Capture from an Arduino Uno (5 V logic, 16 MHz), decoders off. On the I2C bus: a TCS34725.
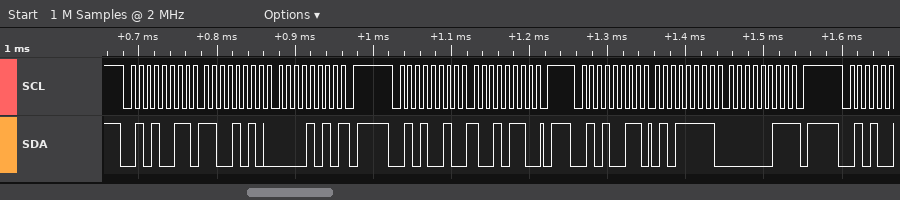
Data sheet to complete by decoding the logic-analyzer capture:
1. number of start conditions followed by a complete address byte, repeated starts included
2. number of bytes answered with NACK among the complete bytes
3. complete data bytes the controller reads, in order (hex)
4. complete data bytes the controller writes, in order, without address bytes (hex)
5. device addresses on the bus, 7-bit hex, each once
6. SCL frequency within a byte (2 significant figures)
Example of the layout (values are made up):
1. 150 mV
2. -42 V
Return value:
1. 3
2. 2
3. CA 0A 5F 03
4. 96
5. 0x29
6. 100 kHz
